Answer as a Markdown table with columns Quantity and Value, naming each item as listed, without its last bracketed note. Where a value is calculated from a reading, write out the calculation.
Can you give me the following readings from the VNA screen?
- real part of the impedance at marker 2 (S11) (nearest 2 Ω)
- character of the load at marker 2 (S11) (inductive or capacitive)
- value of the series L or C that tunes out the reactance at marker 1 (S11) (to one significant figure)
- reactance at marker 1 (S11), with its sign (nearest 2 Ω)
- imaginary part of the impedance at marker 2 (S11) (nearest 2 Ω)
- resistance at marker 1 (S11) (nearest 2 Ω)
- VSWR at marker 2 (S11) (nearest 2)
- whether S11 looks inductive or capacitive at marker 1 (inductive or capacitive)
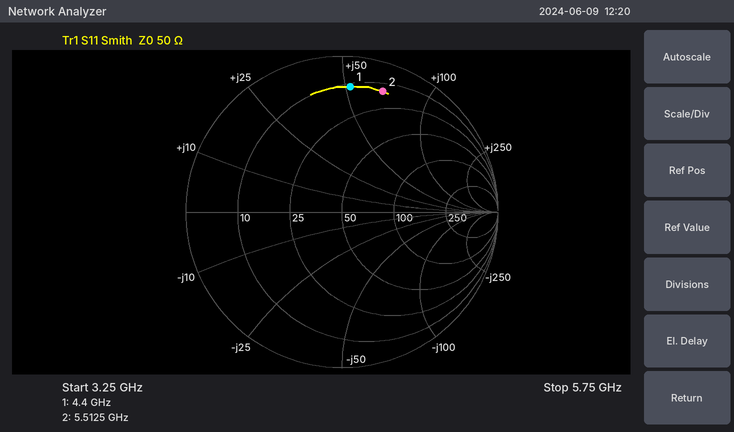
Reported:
| Quantity | Value |
|---|---|
| real part of the impedance at marker 2 (S11) | 14 Ω |
| character of the load at marker 2 (S11) | inductive |
| value of the series L or C that tunes out the reactance at marker 1 (S11) | C = 1/(2π × 4.4 GHz × 52 Ω) ≈ 696 fF, so 700 fF to one significant figure |
| reactance at marker 1 (S11), with its sign | +52 Ω |
| imaginary part of the impedance at marker 2 (S11) | +68 Ω |
| resistance at marker 1 (S11) | 12 Ω |
| VSWR at marker 2 (S11) | 10 |
| whether S11 looks inductive or capacitive at marker 1 | inductive |
